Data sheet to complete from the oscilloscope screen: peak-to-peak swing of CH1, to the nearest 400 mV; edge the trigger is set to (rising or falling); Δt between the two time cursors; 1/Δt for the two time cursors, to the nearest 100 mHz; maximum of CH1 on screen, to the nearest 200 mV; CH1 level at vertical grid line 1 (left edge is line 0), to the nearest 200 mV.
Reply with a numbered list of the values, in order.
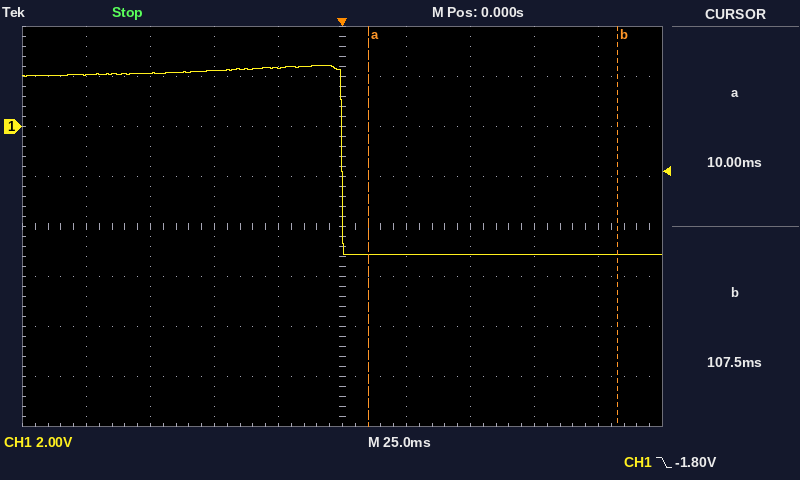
1. 7.6 V
2. falling
3. 97.5 ms
4. 10.3 Hz
5. 2.4 V
6. 2.0 V
